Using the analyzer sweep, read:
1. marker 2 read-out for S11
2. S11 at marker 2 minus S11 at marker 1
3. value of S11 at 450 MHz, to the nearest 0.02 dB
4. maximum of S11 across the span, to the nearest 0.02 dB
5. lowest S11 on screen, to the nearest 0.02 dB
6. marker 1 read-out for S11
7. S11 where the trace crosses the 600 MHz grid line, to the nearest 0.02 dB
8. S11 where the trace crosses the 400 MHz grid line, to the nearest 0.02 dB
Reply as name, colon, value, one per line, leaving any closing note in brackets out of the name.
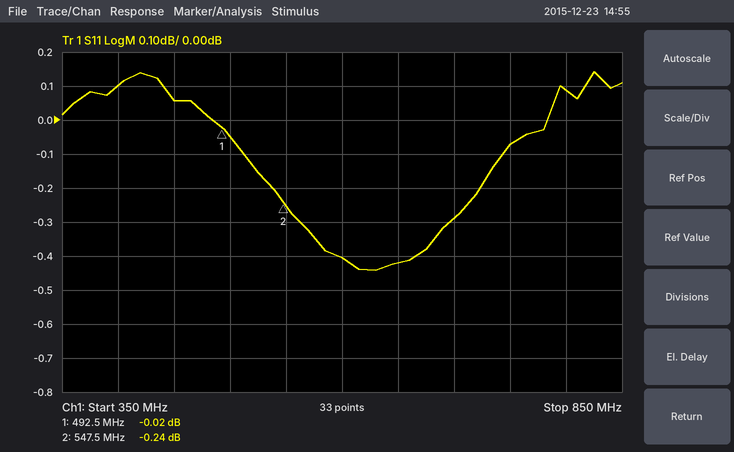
marker 2 read-out for S11: -0.24 dB
S11 at marker 2 minus S11 at marker 1: -0.22 dB
value of S11 at 450 MHz, to the nearest 0.02 dB: 0.06 dB
maximum of S11 across the span, to the nearest 0.02 dB: 0.14 dB
lowest S11 on screen, to the nearest 0.02 dB: -0.44 dB
marker 1 read-out for S11: -0.02 dB
S11 where the trace crosses the 600 MHz grid line, to the nearest 0.02 dB: -0.40 dB
S11 where the trace crosses the 400 MHz grid line, to the nearest 0.02 dB: 0.10 dB
